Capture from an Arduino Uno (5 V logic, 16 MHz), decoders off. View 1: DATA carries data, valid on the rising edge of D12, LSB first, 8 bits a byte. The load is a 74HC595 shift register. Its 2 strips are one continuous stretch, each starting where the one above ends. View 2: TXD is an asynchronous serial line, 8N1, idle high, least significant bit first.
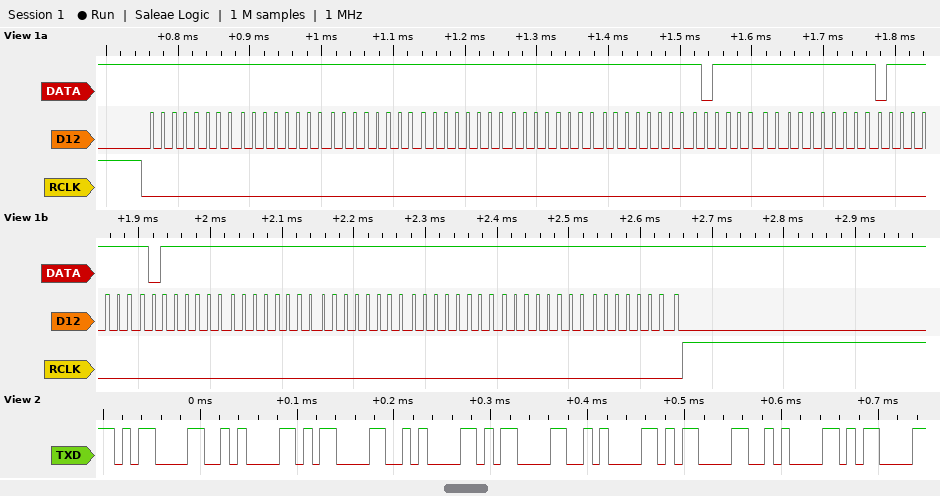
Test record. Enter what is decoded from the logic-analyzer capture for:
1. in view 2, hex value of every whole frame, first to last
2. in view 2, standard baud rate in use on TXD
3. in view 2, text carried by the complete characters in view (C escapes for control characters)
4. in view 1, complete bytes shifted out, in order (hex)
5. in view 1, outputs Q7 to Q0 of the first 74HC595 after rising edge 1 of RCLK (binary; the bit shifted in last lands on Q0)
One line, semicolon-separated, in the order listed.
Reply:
0D 0A 0D 0A 0D 0A 0D 0A 0D; 115200 baud; "\r\n\r\n\r\n\r\n\r"; 0xFF 0xFF 0xFF 0xFF 0xFF 0xFF 0xFD 0xFF 0xFE 0xFD 0xFF 0xFF 0xFF 0xFF 0xFF; 11111111
